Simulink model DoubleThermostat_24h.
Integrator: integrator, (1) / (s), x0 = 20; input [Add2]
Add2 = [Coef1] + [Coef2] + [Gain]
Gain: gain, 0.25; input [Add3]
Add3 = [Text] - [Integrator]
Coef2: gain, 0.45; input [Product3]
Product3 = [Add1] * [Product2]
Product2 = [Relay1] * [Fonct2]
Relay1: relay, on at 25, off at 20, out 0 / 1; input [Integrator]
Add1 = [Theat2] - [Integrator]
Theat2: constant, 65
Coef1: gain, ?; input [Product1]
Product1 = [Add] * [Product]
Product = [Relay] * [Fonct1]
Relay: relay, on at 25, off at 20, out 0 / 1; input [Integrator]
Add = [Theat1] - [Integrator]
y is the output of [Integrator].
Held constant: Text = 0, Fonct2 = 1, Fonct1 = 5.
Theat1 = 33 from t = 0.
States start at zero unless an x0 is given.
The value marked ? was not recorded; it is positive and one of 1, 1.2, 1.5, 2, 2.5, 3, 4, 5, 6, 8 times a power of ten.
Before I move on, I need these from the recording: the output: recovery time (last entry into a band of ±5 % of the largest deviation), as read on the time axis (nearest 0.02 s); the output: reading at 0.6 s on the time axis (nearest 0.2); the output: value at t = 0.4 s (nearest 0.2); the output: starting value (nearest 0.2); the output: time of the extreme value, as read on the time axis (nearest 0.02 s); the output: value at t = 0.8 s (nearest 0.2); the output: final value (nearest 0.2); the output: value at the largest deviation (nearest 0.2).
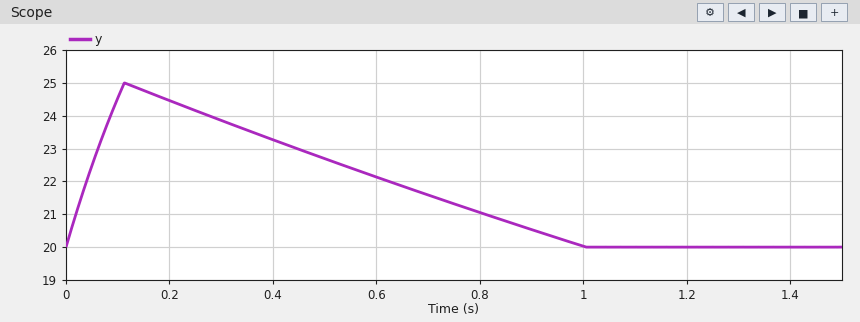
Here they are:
0.96 s
22.2
23.2
20.0
0.12 s
21.0
20.0
25.0
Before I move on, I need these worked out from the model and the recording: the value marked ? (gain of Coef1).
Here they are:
0.6
